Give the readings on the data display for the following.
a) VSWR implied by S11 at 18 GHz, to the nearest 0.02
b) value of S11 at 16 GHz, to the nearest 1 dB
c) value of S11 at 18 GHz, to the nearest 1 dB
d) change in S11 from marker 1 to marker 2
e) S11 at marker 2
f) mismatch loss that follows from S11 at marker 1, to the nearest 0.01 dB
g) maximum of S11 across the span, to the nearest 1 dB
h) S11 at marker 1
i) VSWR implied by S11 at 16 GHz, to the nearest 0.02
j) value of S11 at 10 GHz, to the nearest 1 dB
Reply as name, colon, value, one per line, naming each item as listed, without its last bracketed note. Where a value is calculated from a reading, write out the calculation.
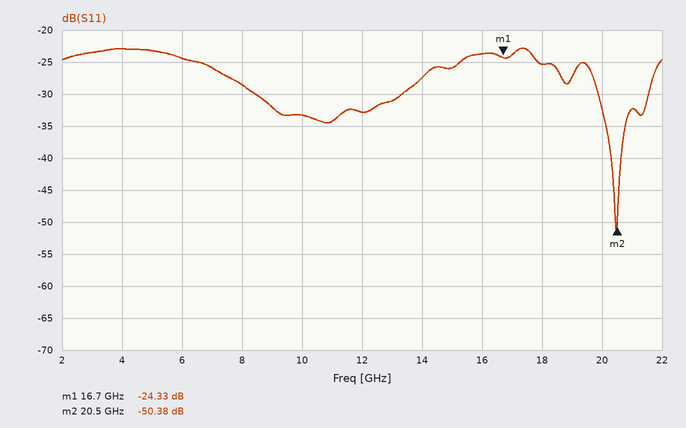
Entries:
VSWR implied by S11 at 18 GHz, to the nearest 0.02: |Γ| = 10^(-25/20) = 0.0562; VSWR = (1 + 0.0562)/(1 − 0.0562) ≈ 1.12
value of S11 at 16 GHz, to the nearest 1 dB: -24 dB
value of S11 at 18 GHz, to the nearest 1 dB: -25 dB
change in S11 from marker 1 to marker 2: -50.38 − (-24.33) = -26.05 dB
S11 at marker 2: -50.38 dB
mismatch loss that follows from S11 at marker 1, to the nearest 0.01 dB: −10 log10(1 − 10^(-24.33/10)) ≈ 0.02 dB
maximum of S11 across the span, to the nearest 1 dB: -23 dB
S11 at marker 1: -24.33 dB
VSWR implied by S11 at 16 GHz, to the nearest 0.02: |Γ| = 10^(-24/20) = 0.0631; VSWR = (1 + 0.0631)/(1 − 0.0631) ≈ 1.13, so 1.14 to the nearest 0.02
value of S11 at 10 GHz, to the nearest 1 dB: -33 dB
